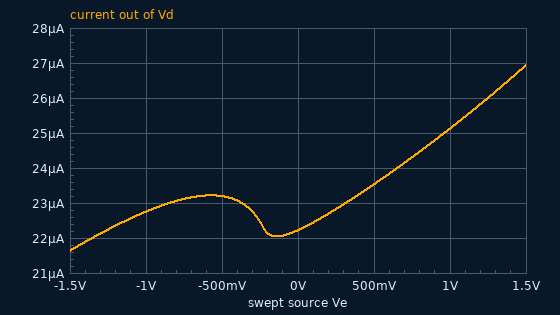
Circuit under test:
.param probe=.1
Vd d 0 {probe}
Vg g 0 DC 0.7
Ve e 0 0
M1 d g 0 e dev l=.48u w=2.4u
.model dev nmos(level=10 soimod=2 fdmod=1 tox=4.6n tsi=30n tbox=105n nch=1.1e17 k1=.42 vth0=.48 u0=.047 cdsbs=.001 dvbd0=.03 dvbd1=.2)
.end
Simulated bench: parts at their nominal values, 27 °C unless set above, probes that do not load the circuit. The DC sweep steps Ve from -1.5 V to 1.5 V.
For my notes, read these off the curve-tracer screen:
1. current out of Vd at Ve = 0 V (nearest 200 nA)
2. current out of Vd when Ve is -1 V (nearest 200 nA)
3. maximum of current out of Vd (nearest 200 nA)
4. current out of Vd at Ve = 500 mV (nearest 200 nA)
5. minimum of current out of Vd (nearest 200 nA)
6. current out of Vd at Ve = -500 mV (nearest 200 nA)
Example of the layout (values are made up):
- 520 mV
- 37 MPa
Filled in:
- 22.2 µA
- 22.8 µA
- 27.0 µA
- 23.6 µA
- 21.6 µA
- 23.2 µA
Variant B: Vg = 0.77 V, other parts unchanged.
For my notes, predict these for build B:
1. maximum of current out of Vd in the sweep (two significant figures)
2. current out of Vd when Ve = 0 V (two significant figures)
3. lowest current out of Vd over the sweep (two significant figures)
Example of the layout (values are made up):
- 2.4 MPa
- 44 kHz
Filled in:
- 34 µA
- 29 µA
- 28 µA
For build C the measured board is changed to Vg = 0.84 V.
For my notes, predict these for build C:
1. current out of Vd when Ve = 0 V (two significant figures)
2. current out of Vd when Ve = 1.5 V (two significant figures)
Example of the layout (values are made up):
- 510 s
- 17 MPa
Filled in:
- 35 µA
- 40 µA
